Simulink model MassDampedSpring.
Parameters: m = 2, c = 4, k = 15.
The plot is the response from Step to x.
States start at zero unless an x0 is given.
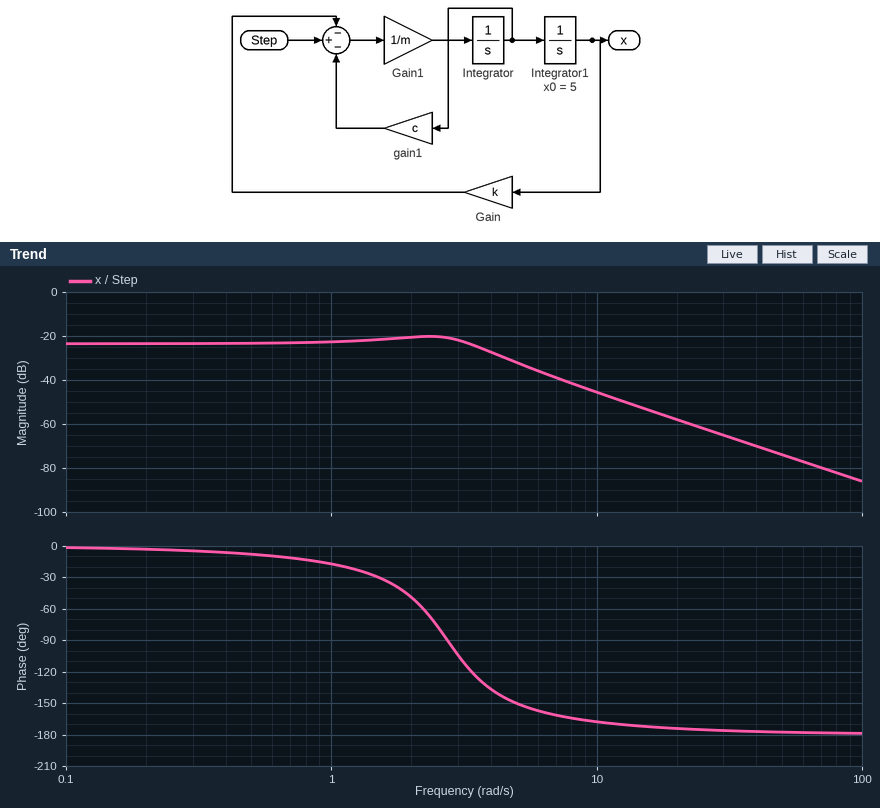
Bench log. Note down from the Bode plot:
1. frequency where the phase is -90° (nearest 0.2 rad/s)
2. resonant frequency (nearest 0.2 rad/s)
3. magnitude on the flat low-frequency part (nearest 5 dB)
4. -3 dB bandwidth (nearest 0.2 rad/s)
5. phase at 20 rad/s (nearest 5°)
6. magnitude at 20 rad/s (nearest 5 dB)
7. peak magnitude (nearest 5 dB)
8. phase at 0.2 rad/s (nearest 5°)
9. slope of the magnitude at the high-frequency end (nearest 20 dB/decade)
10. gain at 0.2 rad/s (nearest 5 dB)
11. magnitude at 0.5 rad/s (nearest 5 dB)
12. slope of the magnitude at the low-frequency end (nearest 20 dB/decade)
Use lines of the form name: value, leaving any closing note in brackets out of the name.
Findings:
frequency where the phase is -90°: 2.8 rad/s
resonant frequency: 2.4 rad/s
magnitude on the flat low-frequency part: -25 dB
-3 dB bandwidth: 3.8 rad/s
phase at 20 rad/s: -175°
magnitude at 20 rad/s: -60 dB
peak magnitude: -20 dB
phase at 0.2 rad/s: -5°
slope of the magnitude at the high-frequency end: -40 dB/decade
gain at 0.2 rad/s: -25 dB
magnitude at 0.5 rad/s: -25 dB
slope of the magnitude at the low-frequency end: 0 dB/decade
